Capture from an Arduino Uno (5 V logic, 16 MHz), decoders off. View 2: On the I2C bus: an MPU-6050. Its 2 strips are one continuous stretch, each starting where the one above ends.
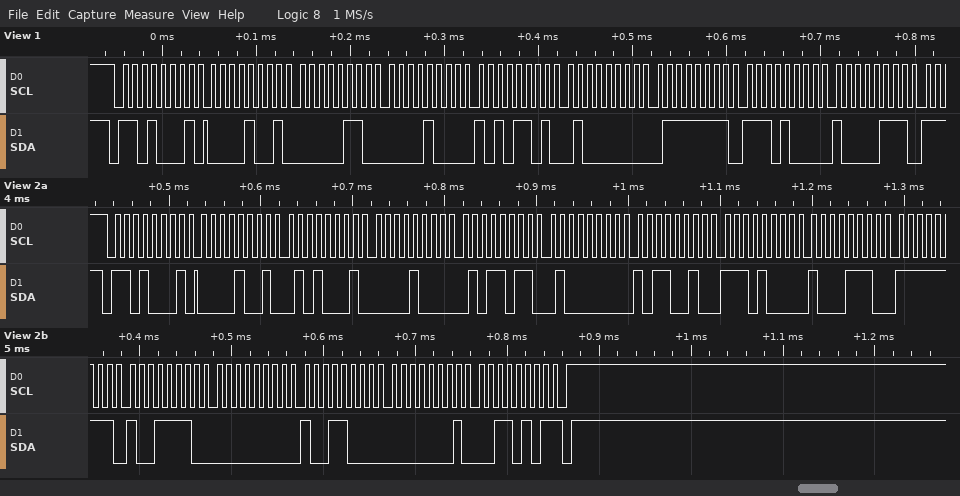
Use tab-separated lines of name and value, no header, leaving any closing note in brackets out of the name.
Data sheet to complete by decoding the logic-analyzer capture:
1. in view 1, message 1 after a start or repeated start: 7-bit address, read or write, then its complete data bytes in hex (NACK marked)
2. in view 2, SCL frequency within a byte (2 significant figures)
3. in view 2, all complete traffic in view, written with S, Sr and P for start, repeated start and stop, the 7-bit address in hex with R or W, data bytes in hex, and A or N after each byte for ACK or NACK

in view 1, message 1 after a start or repeated start: 7-bit address, read or write, then its complete data bytes in hex	0x68 read: 09 06 08 AD 40 7F E8 87
in view 2, SCL frequency within a byte	100 kHz
in view 2, all complete traffic in view, written with S, Sr and P for start, repeated start and stop, the 7-bit address in hex with R or W, data bytes in hex, and A or N after each byte for ACK or NACK	S 68R A 09 A 51 A 08 A 5B A 40 A B2 A E8 A 8E A FF A 9E A 00 A 98 A 01 A 35 N P
